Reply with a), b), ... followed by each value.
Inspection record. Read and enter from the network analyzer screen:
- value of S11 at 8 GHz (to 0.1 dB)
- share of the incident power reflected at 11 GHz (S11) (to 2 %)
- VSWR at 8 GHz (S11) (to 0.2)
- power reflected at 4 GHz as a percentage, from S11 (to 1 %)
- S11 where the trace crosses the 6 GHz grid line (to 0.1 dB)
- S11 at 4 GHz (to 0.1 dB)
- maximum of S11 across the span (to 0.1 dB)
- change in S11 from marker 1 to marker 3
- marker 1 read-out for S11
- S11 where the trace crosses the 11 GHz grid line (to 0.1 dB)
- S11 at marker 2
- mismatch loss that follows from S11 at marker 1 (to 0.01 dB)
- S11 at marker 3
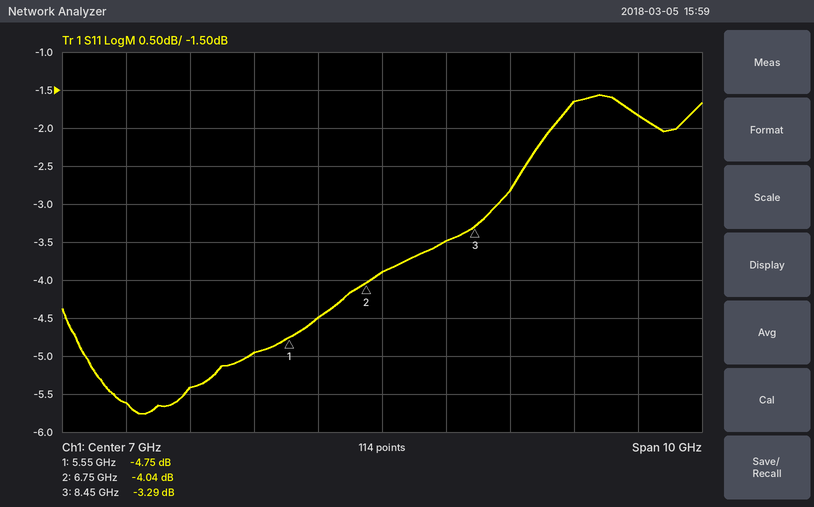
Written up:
a) -3.5 dB
b) 66 %
c) 5.0
d) 29 %
e) -4.5 dB
f) -5.4 dB
g) -1.6 dB
h) 1.46 dB
i) -4.75 dB
j) -1.8 dB
k) -4.04 dB
l) 1.77 dB
m) -3.29 dB
